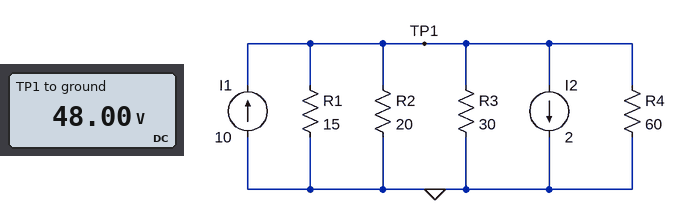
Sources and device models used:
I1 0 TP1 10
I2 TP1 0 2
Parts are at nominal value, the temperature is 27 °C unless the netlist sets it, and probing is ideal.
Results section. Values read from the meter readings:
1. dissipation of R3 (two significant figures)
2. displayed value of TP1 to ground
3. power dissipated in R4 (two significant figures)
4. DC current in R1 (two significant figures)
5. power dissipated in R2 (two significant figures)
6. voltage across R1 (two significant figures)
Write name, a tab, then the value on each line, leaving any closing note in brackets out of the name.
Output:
dissipation of R3	77 W
displayed value of TP1 to ground	48.00 V
power dissipated in R4	38 W
DC current in R1	3.2 A
power dissipated in R2	120 W
voltage across R1	48 V
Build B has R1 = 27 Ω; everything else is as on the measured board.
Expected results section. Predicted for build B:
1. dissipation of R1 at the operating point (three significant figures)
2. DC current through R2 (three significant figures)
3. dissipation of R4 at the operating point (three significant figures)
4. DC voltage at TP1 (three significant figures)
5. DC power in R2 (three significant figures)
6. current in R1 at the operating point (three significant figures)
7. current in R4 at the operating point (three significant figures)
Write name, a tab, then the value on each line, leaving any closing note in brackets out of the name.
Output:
dissipation of R1 at the operating point	126 W
DC current through R2	2.92 A
dissipation of R4 at the operating point	56.8 W
DC voltage at TP1	58.4 V
DC power in R2	170 W
current in R1 at the operating point	2.16 A
current in R4 at the operating point	973 mA
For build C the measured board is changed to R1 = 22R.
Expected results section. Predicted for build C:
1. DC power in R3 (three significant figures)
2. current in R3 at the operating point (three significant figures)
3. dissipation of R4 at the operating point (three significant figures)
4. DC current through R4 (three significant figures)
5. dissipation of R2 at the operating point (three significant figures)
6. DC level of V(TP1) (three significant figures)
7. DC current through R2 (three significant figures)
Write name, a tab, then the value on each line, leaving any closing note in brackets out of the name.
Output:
DC power in R3	101 W
current in R3 at the operating point	1.83 A
dissipation of R4 at the operating point	50.4 W
DC current through R4	917 mA
dissipation of R2 at the operating point	151 W
DC level of V(TP1)	55.0 V
DC current through R2	2.75 A
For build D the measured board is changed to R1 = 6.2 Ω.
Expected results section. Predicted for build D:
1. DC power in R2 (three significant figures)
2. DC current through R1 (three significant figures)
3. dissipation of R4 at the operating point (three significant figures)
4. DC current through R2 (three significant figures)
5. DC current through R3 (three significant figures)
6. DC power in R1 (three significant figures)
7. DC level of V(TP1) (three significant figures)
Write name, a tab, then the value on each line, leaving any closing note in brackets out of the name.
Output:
DC power in R2	46.9 W
DC current through R1	4.94 A
dissipation of R4 at the operating point	15.6 W
DC current through R2	1.53 A
DC current through R3	1.02 A
DC power in R1	151 W
DC level of V(TP1)	30.6 V
